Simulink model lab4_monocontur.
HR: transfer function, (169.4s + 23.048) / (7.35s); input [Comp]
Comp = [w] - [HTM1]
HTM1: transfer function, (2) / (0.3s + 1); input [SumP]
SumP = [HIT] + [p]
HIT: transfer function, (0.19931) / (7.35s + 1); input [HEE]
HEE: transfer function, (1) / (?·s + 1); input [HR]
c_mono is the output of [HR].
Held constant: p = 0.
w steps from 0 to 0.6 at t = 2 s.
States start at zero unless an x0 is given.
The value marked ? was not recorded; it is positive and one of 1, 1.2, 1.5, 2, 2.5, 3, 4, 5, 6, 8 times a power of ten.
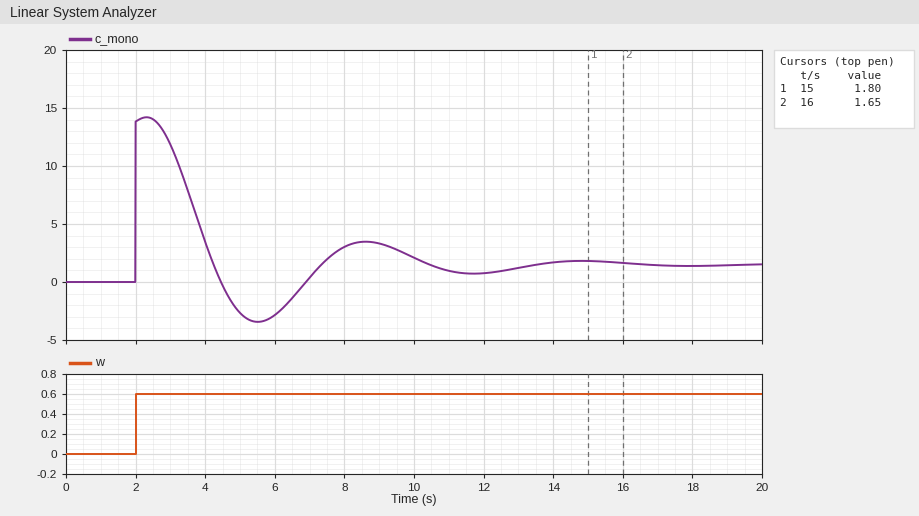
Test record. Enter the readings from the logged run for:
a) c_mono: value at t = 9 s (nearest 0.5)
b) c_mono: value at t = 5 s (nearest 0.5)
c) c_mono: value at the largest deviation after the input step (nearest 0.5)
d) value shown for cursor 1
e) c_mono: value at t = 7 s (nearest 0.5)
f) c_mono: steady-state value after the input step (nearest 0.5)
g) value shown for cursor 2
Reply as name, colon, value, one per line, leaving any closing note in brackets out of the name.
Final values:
c_mono: value at t = 9 s: 3.5
c_mono: value at t = 5 s: -2.5
c_mono: value at the largest deviation after the input step: 14.0
value shown for cursor 1: 1.80
c_mono: value at t = 7 s: 0.5
c_mono: steady-state value after the input step: 1.5
value shown for cursor 2: 1.65
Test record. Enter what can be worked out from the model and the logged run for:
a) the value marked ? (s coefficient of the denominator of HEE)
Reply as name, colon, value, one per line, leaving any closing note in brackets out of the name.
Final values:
the value marked ?: 1
